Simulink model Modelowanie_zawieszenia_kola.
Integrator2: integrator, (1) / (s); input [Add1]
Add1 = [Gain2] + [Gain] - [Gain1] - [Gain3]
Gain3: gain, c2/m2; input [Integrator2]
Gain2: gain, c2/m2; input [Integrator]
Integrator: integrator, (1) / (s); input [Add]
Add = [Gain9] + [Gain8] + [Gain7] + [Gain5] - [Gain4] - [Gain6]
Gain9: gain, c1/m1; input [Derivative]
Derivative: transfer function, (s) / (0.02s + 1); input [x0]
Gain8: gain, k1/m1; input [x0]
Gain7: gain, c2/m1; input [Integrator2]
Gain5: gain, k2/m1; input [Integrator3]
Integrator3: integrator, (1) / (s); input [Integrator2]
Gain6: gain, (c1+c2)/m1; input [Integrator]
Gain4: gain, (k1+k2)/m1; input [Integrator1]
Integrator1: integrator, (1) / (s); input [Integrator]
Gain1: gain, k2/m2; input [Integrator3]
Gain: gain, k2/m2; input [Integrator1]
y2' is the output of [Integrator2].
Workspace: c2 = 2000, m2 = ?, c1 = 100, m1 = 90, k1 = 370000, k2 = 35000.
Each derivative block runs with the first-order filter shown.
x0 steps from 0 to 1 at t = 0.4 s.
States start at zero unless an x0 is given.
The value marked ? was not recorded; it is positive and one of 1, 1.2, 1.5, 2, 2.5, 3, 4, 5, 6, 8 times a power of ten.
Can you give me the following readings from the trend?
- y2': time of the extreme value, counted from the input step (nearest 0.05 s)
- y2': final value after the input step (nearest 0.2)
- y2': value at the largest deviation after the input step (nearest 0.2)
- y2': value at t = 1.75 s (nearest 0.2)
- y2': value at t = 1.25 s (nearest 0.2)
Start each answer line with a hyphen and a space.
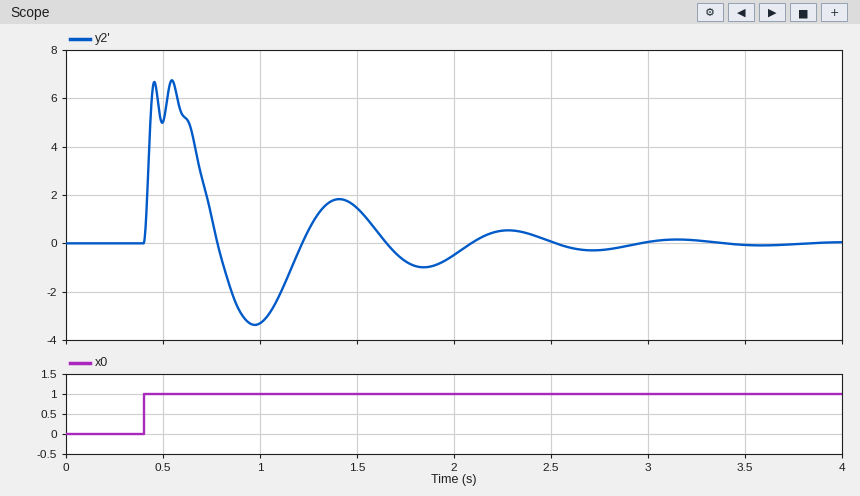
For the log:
- 0.15 s
- 0.0
- 6.8
- -0.8
- 0.6
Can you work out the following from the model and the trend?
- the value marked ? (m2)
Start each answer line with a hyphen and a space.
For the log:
- 600
